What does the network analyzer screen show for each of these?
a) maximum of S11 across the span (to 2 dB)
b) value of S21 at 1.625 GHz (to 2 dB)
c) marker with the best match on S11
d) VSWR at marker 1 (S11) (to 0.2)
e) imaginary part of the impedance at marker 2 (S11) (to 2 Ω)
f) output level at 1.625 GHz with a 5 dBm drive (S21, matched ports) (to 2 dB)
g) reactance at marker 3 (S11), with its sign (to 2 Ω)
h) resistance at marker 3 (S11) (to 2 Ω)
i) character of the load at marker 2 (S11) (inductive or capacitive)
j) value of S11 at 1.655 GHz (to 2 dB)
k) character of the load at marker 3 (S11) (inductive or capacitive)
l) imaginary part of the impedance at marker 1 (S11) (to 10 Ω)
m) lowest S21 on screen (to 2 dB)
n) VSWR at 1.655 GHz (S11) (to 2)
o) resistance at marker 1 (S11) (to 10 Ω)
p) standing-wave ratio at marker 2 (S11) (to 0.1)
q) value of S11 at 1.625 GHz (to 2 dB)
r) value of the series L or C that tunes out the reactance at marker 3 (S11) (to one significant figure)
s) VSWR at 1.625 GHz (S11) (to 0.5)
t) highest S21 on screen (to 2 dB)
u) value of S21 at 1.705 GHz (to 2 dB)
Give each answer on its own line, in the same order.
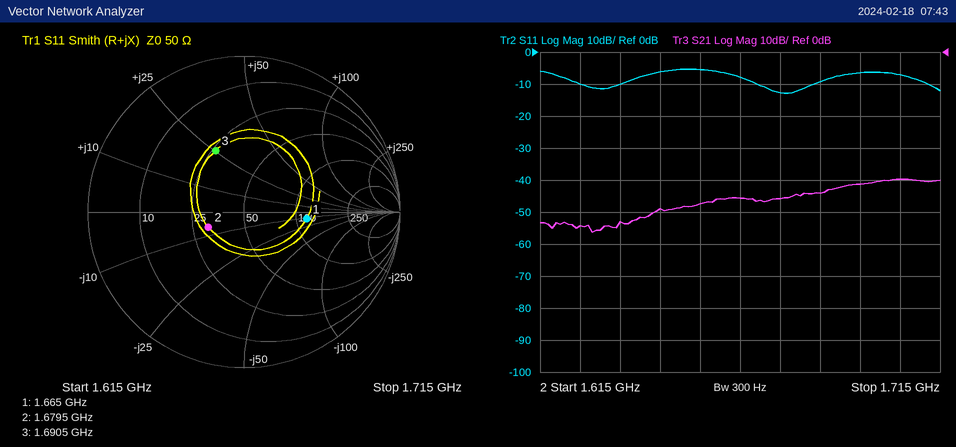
-6 dB
-54 dB
marker 2
2.4
-6 Ω
-50 dBm
+26 Ω
26 Ω
capacitive
-6 dB
inductive
-10 Ω
-56 dB
4
120 Ω
1.7
-10 dB
4 pF
2.0
-40 dB
-40 dB
